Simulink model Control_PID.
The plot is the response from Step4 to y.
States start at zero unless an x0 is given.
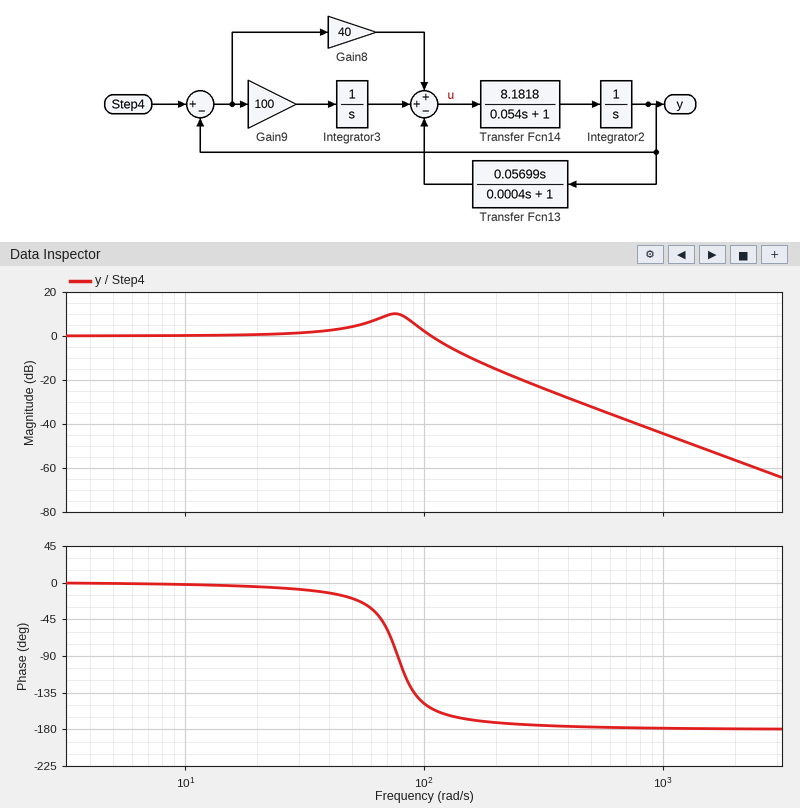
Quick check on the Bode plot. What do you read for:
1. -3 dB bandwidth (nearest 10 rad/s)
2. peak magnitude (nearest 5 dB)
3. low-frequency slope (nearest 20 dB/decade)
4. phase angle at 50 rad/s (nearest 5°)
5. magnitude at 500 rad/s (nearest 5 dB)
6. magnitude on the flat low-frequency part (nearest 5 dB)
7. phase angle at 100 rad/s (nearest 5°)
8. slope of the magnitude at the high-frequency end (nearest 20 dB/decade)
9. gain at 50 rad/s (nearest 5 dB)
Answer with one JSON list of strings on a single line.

["120 rad/s", "10 dB", "0 dB/decade", "-20°", "-30 dB", "0 dB", "-150°", "-40 dB/decade", "5 dB"]
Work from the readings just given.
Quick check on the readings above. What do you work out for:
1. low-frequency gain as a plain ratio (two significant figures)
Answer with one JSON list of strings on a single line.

["1.0"]
